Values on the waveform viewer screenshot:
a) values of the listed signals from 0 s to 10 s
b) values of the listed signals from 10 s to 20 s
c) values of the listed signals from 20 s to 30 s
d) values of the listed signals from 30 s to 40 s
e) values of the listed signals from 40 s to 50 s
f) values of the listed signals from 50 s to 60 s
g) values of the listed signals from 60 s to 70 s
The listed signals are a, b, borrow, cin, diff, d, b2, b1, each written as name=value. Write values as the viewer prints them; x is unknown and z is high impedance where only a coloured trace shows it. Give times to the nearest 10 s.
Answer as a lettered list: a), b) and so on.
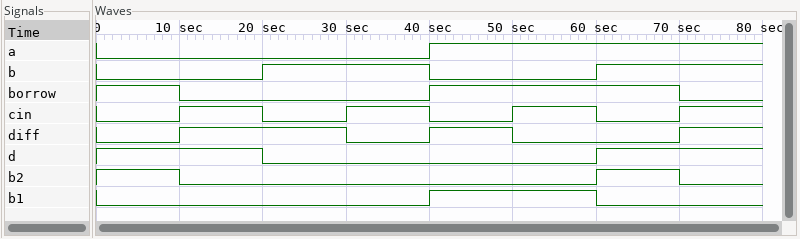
a) a=0, b=0, borrow=1, cin=0, diff=0, d=1, b2=1, b1=0
b) a=0, b=0, borrow=0, cin=1, diff=1, d=1, b2=0, b1=0
c) a=0, b=1, borrow=0, cin=0, diff=1, d=0, b2=0, b1=0
d) a=0, b=1, borrow=0, cin=1, diff=0, d=0, b2=0, b1=0
e) a=1, b=0, borrow=1, cin=0, diff=1, d=0, b2=0, b1=1
f) a=1, b=0, borrow=1, cin=1, diff=0, d=0, b2=0, b1=1
g) a=1, b=1, borrow=1, cin=0, diff=0, d=1, b2=1, b1=0
